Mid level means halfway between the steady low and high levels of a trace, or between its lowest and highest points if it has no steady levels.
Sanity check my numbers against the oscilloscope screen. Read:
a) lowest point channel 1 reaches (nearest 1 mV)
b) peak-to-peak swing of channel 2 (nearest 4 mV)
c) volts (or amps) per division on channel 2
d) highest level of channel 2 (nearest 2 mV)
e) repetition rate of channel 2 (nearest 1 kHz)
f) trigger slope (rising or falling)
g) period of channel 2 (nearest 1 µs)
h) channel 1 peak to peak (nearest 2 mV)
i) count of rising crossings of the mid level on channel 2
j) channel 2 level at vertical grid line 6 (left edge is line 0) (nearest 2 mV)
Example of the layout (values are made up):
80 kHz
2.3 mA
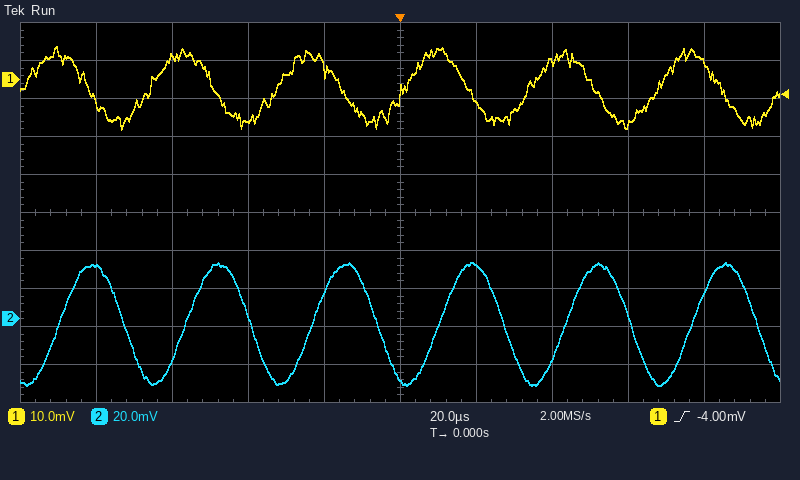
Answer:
-13 mV
64 mV
20 mV
30 mV
30 kHz
rising
33 µs
22 mV
6
28 mV
